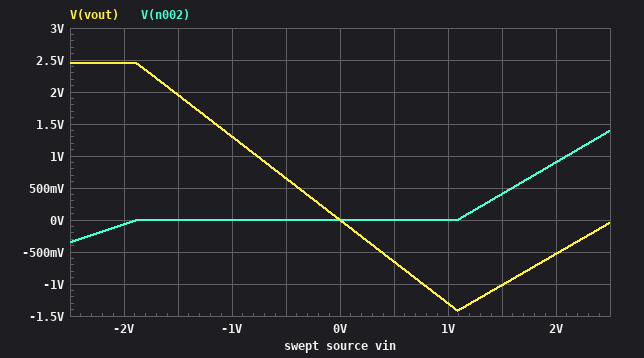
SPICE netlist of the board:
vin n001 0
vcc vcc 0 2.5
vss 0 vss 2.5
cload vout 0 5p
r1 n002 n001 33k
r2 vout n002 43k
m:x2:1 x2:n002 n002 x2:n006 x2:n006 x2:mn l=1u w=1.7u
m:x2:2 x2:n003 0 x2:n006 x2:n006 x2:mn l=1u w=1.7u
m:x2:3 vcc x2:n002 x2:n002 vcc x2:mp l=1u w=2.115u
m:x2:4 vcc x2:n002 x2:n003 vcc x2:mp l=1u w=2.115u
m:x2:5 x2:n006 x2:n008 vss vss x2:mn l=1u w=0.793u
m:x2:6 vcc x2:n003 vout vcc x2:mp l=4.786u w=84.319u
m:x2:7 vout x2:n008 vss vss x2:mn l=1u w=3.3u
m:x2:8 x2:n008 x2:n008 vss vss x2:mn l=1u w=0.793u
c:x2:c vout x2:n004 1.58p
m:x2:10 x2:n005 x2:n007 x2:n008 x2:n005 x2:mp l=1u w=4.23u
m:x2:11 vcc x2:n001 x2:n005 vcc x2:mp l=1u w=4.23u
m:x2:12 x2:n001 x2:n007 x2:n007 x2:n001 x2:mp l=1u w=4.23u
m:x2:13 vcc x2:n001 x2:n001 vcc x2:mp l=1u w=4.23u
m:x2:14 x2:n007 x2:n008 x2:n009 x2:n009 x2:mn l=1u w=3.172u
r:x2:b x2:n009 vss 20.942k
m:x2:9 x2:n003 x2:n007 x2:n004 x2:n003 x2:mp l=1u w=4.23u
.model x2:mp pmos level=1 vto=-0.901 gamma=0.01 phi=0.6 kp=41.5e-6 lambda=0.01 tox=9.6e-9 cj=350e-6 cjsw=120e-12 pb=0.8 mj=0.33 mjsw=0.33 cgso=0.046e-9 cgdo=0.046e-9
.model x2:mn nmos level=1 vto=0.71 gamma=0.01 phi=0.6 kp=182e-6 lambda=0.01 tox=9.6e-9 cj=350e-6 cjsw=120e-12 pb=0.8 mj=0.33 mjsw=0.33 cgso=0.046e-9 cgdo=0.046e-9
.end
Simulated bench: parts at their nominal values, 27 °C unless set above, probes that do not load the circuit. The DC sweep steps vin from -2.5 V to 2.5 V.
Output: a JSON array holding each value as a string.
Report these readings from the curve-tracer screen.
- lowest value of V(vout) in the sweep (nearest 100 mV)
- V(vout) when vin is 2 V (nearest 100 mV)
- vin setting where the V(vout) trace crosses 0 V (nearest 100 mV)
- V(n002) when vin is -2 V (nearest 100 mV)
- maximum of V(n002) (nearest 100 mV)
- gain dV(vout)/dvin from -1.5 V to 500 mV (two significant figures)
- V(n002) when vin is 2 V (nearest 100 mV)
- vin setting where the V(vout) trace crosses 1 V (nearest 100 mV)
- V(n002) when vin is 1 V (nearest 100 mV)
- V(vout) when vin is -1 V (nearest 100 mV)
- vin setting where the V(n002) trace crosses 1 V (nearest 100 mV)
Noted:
["-1.4 V", "-500 mV", "0 V", "-100 mV", "1.4 V", "-1.3 V/V", "900 mV", "-800 mV", "0 V", "1.3 V", "2.1 V"]
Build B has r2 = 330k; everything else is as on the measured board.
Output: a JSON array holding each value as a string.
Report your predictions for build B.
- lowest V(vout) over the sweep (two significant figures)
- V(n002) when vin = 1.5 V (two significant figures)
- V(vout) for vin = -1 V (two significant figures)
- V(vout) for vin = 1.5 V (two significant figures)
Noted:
["-2.5 V", "1.1 V", "2.5 V", "-2.4 V"]
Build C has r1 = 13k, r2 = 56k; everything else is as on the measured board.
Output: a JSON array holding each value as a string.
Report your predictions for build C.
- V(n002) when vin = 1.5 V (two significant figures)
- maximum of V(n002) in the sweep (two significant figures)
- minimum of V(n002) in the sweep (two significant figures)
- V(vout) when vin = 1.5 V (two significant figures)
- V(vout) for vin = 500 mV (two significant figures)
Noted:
["1.1 V", "2.1 V", "-1.6 V", "-790 mV", "-1.8 V"]
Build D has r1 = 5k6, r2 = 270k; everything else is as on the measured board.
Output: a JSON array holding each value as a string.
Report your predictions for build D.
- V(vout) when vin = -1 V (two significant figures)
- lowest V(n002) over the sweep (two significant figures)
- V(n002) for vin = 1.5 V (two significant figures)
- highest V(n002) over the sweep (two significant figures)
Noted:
["2.5 V", "-2.4 V", "1.4 V", "2.4 V"]
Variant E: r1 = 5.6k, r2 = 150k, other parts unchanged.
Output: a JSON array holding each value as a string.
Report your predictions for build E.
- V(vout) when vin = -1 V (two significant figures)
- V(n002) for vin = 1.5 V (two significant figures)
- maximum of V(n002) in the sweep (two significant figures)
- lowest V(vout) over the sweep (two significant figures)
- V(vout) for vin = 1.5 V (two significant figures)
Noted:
["2.5 V", "1.4 V", "2.3 V", "-2.4 V", "-2.3 V"]
